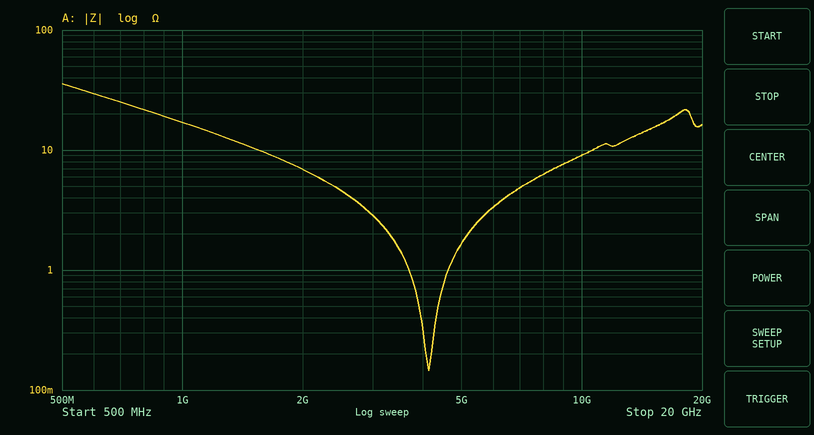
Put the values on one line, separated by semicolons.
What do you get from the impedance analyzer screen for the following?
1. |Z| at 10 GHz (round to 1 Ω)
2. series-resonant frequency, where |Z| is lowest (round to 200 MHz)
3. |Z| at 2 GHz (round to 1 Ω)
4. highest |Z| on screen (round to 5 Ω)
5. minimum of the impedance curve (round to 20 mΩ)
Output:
9 Ω; 4.2 GHz; 7 Ω; 35 Ω; 140 mΩ
